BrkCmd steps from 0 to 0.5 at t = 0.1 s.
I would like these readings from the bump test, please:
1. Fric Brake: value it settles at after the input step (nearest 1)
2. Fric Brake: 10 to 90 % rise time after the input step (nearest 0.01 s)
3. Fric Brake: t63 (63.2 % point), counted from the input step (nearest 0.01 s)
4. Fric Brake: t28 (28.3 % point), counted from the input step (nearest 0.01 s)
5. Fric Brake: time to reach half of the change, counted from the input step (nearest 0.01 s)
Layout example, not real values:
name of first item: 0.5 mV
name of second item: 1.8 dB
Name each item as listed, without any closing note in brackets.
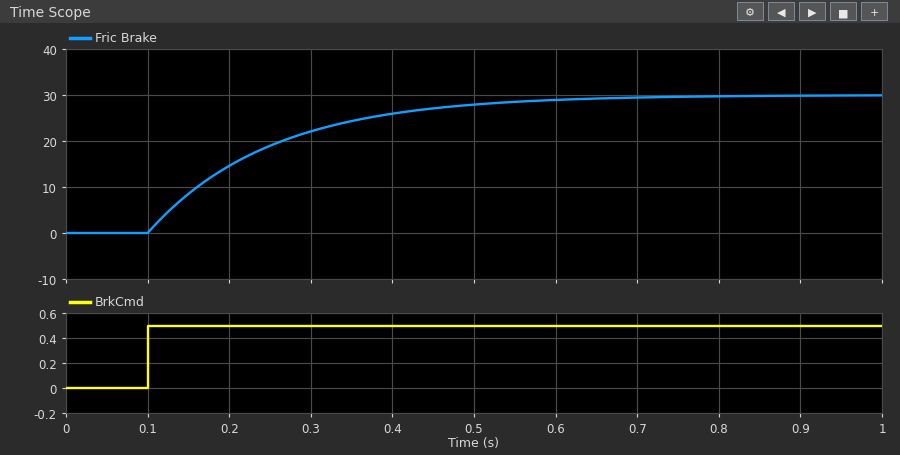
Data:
Fric Brake: value it settles at after the input step: 30
Fric Brake: 10 to 90 % rise time after the input step: 0.33 s
Fric Brake: t63 (63.2 % point), counted from the input step: 0.15 s
Fric Brake: t28 (28.3 % point), counted from the input step: 0.05 s
Fric Brake: time to reach half of the change, counted from the input step: 0.10 s
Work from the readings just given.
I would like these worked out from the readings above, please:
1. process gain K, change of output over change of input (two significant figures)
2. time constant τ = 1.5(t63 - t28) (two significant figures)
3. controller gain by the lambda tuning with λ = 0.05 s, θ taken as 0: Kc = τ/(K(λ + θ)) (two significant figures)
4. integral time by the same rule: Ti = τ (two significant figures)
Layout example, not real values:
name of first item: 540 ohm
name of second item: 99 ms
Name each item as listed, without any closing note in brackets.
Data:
process gain K, change of output over change of input: 60
time constant τ = 1.5(t63 - t28): 0.15 s
controller gain by the lambda tuning with λ = 0.05 s, θ taken as 0: Kc = τ/(K(λ + θ)): 0.050
integral time by the same rule: Ti = τ: 0.15 s
